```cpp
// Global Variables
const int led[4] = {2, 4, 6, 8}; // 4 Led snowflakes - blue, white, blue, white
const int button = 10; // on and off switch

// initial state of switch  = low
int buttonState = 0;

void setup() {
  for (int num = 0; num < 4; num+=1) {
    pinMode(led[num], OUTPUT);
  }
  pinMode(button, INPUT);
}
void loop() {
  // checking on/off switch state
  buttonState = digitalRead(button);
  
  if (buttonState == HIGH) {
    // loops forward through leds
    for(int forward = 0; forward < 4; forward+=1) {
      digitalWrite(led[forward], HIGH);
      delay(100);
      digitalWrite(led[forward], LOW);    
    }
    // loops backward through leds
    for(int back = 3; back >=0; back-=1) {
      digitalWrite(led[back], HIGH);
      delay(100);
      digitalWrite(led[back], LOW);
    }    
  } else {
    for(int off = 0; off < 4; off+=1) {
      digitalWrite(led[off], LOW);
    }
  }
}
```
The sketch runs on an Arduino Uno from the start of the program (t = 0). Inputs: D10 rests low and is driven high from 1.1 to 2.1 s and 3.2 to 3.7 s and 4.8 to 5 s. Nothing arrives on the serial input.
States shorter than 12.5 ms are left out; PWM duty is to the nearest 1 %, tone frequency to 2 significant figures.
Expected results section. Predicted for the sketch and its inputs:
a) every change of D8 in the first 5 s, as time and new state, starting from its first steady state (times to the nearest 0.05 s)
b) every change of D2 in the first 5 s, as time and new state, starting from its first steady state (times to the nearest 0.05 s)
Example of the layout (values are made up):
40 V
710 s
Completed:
0 s low; 1.4 s high; 1.6 s low; 2.2 s high; 2.4 s low; 3.5 s high; 3.7 s low
0 s low; 1.1 s high; 1.2 s low; 1.8 s high; 2 s low; 2.6 s high; 2.7 s low; 3.2 s high; 3.3 s low; 3.9 s high; 4 s low; 4.8 s high; 4.9 s low
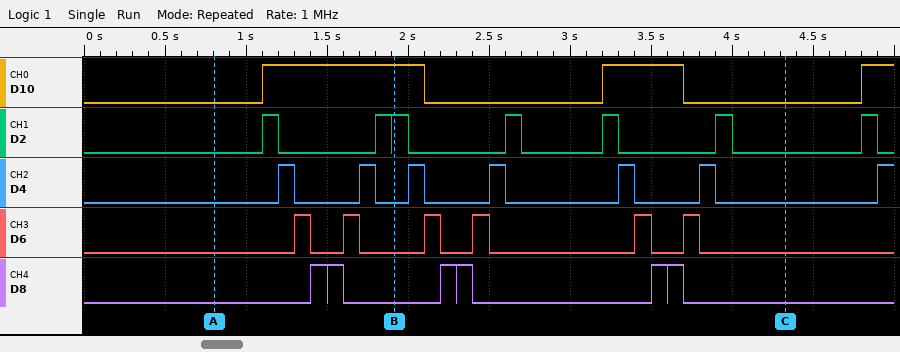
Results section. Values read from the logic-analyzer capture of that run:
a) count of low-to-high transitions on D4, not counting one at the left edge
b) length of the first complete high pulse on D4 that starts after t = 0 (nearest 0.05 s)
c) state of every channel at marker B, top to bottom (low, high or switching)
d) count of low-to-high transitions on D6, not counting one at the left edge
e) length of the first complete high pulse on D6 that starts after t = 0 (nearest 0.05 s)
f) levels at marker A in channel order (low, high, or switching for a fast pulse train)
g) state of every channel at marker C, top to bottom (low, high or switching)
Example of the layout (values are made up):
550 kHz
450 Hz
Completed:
7
0.10 s
D10 high, D2 high, D4 low, D6 low, D8 low
6
0.10 s
D10 low, D2 low, D4 low, D6 low, D8 low
D10 low, D2 low, D4 low, D6 low, D8 low
